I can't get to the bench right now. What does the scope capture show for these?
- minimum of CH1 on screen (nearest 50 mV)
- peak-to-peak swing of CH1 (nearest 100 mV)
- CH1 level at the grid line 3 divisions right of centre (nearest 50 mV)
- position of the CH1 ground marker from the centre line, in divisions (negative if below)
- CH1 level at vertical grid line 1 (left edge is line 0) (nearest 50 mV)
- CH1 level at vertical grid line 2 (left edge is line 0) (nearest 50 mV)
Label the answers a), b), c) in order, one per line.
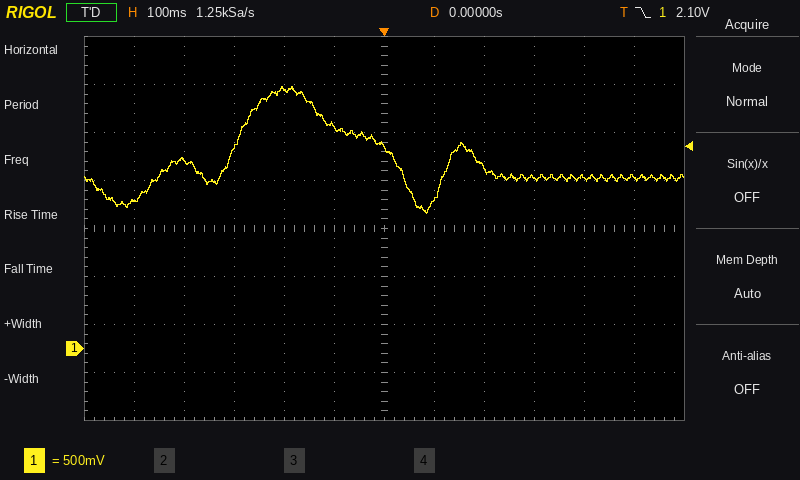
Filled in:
a) 1.40 V
b) 1.30 V
c) 1.80 V
d) -2.5 div
e) 1.55 V
f) 1.95 V
